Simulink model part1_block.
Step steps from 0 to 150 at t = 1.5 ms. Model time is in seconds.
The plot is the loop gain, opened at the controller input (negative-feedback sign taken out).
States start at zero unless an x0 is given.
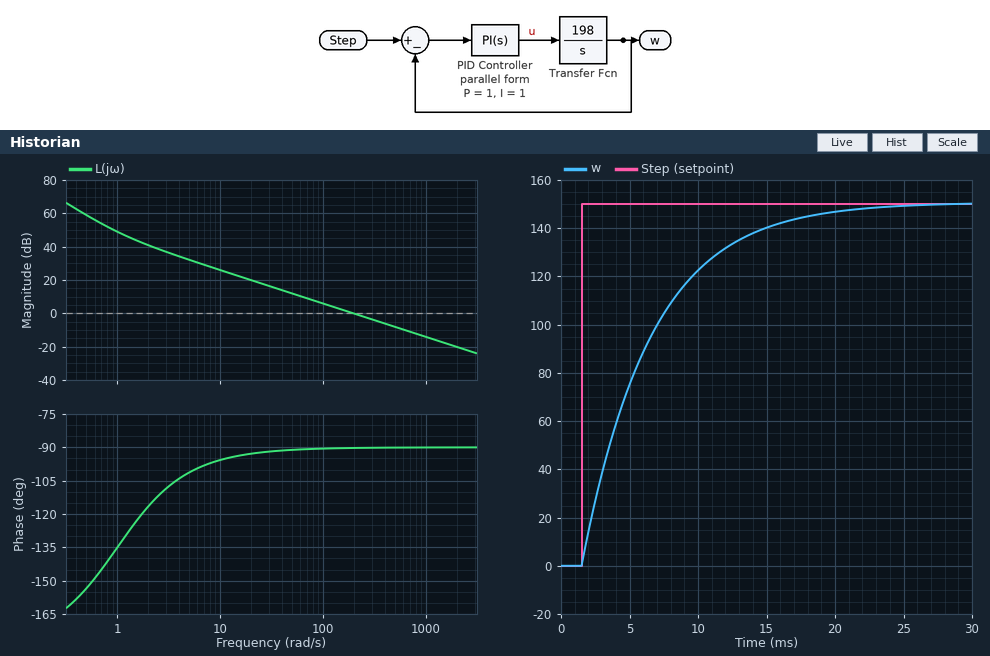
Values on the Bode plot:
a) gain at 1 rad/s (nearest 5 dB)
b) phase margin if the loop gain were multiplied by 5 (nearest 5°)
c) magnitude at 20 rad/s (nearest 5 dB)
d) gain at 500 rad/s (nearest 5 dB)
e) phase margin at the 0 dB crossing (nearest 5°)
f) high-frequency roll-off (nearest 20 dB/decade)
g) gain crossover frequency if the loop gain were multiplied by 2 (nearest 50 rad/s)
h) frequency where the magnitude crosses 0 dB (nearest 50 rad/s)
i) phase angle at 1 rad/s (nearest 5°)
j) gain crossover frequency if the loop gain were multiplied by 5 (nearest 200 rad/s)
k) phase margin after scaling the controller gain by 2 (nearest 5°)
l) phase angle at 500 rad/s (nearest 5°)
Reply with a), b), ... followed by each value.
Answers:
a) 50 dB
b) 90°
c) 20 dB
d) -10 dB
e) 90°
f) -20 dB/decade
g) 400 rad/s
h) 200 rad/s
i) -135°
j) 1000 rad/s
k) 90°
l) -90°
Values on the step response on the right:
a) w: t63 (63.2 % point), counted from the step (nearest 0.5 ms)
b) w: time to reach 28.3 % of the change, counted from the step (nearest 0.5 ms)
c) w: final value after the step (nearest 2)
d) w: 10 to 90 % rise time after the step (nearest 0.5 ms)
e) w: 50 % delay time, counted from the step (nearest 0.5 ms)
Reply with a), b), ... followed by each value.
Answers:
a) 5.0 ms
b) 1.5 ms
c) 150
d) 11.0 ms
e) 3.5 ms
